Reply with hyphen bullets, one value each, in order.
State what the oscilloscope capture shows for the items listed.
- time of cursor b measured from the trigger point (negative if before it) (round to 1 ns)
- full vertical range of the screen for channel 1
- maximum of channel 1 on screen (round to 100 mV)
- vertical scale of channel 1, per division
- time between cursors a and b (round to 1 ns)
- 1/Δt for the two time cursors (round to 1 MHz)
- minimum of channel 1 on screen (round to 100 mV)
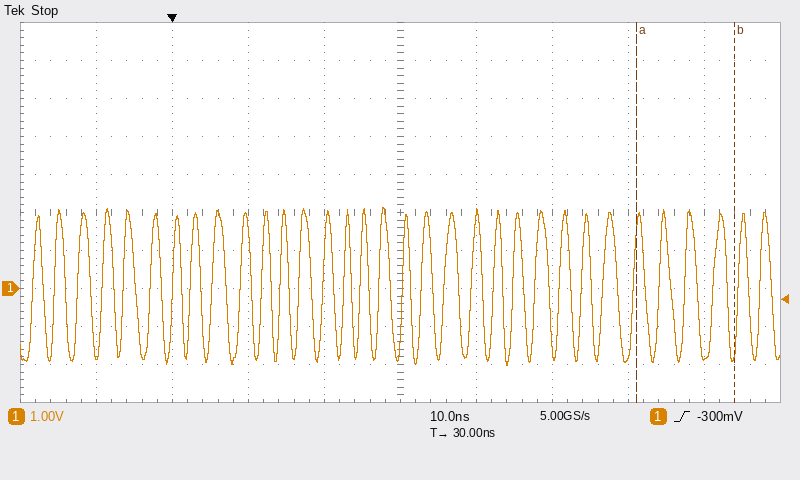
- +74 ns
- 10 V
- 2.1 V
- 1 V
- 13 ns
- 77 MHz
- -2.0 V
